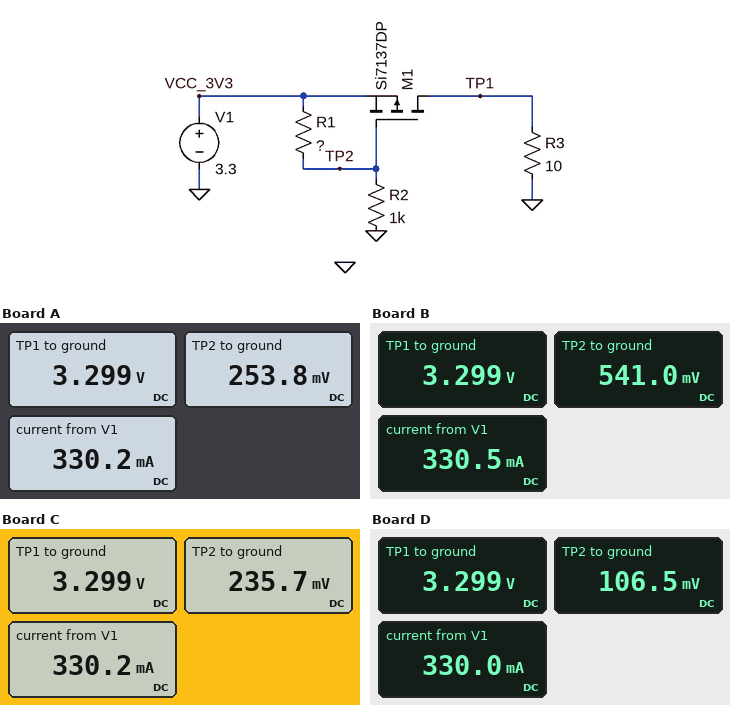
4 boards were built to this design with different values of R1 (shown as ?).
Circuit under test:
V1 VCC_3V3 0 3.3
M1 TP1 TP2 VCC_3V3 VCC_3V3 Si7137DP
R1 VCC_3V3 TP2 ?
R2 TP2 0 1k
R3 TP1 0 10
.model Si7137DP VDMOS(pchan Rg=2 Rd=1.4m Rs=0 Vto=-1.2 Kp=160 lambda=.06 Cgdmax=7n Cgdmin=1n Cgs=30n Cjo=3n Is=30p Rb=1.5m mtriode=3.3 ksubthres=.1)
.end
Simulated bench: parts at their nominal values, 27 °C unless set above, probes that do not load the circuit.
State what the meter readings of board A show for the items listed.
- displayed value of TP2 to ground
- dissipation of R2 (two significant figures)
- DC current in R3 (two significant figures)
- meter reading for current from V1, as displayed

253.8 mV
64 µW
330 mA
330.2 mA
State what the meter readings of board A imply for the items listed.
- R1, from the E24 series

12 kΩ
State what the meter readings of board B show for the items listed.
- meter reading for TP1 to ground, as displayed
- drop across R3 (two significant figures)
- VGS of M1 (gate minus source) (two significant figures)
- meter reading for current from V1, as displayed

3.299 V
3.3 V
-2.8 V
330.5 mA
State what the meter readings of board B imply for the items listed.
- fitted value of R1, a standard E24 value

5.1 kΩ
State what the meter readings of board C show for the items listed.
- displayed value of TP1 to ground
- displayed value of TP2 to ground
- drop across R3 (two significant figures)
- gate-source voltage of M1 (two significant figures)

3.299 V
235.7 mV
3.3 V
-3.1 V
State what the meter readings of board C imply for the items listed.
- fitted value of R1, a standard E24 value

13 kΩ
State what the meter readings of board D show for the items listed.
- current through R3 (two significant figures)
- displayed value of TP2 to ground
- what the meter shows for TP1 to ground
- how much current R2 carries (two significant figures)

330 mA
106.5 mV
3.299 V
110 µA
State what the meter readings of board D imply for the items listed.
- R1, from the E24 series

30 kΩ
